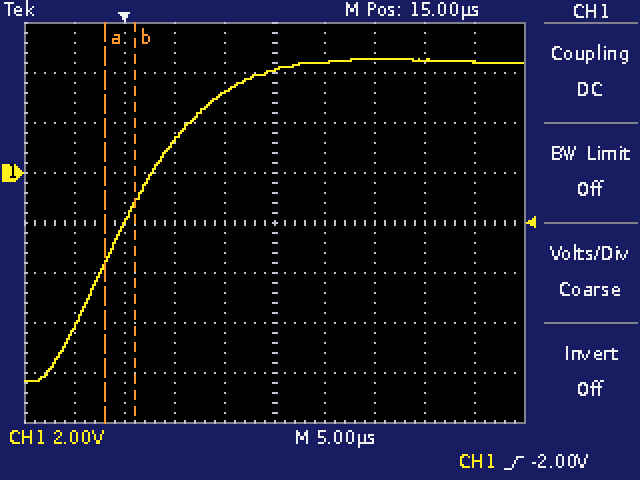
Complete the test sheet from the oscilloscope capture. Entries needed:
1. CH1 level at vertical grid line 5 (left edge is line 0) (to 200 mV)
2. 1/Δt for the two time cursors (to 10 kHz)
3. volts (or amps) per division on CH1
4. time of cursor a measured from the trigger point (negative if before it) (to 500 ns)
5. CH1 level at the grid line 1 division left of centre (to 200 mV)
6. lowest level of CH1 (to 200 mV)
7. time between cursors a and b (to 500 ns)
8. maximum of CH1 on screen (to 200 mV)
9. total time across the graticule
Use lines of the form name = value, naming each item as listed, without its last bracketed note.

CH1 level at vertical grid line 5 (left edge is line 0) = 4.2 V
1/Δt for the two time cursors = 330 kHz
volts (or amps) per division on CH1 = 2 V
time of cursor a measured from the trigger point (negative if before it) = -2.0 µs
CH1 level at the grid line 1 division left of centre = 3.2 V
lowest level of CH1 = -8.4 V
time between cursors a and b = 3.0 µs
maximum of CH1 on screen = 4.6 V
total time across the graticule = 50 µs
